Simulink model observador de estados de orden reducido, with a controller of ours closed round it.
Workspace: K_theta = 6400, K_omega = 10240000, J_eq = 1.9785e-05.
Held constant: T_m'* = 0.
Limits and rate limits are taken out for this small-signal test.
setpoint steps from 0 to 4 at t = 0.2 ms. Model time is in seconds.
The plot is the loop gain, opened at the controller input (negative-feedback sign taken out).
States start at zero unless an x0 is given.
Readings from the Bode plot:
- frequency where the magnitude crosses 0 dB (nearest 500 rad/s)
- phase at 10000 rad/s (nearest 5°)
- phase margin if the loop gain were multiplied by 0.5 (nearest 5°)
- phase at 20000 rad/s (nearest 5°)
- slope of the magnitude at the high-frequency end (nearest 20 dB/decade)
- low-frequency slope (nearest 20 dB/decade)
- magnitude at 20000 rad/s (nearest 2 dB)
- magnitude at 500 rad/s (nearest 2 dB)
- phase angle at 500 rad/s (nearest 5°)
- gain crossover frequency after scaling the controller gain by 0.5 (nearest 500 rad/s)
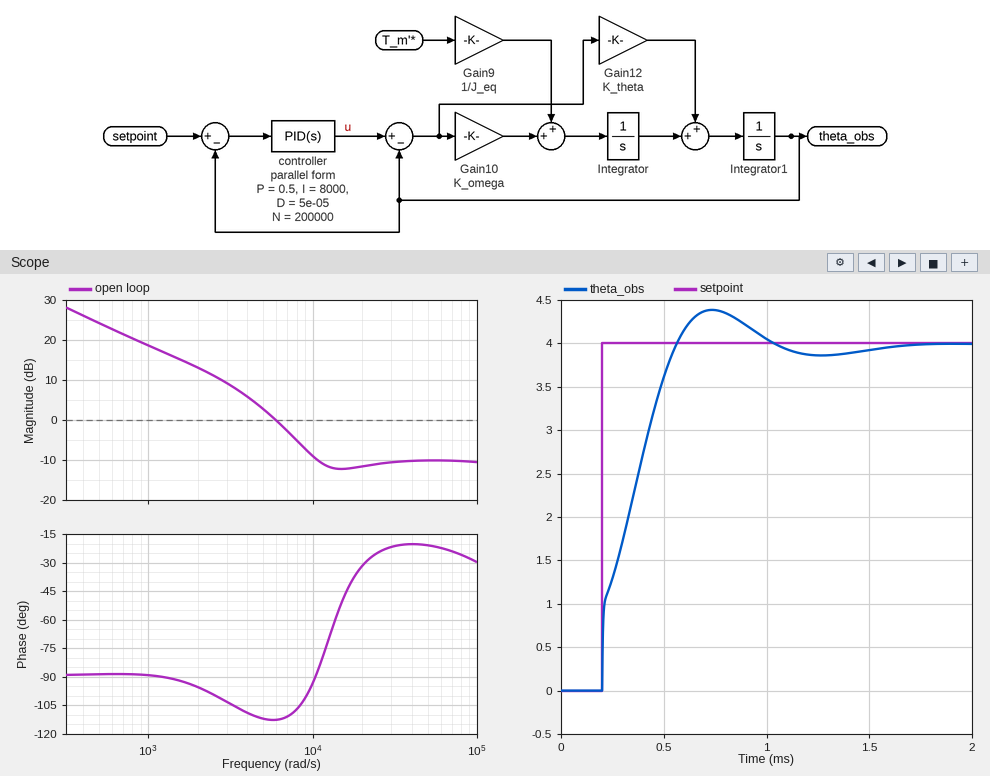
6000 rad/s
-95°
70°
-30°
0 dB/decade
-20 dB/decade
-12 dB
24 dB
-90°
4000 rad/s
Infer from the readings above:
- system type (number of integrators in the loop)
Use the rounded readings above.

1
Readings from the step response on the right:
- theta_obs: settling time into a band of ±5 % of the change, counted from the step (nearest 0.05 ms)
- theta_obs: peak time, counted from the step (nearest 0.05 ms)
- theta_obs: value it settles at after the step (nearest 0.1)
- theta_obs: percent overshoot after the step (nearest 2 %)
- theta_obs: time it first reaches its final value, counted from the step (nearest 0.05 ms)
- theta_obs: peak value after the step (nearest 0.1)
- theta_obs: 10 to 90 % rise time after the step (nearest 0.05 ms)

0.70 ms
0.55 ms
4.0
10 %
0.35 ms
4.4
0.30 ms
